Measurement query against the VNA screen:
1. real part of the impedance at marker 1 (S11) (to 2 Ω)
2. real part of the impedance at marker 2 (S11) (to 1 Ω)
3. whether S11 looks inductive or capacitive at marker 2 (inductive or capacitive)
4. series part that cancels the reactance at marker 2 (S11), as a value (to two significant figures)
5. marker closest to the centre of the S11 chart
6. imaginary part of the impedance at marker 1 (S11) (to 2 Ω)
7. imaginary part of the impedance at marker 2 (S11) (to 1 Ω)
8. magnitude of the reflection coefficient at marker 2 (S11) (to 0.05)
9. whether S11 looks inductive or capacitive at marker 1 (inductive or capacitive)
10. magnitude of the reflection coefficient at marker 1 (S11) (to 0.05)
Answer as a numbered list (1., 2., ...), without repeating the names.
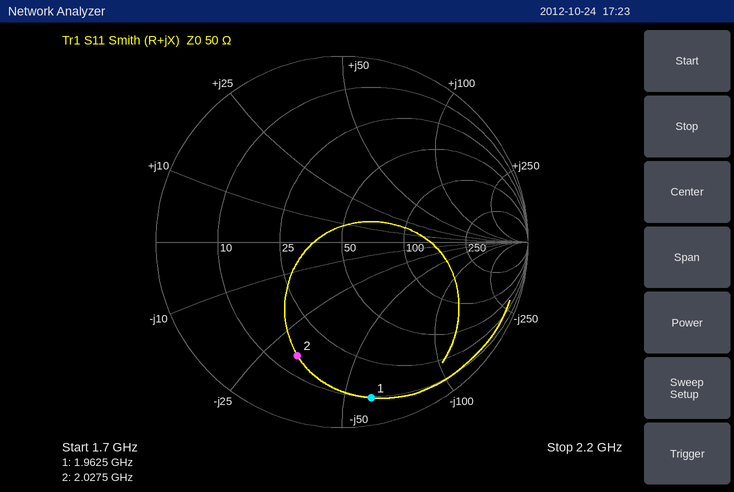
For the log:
1. 10 Ω
2. 15 Ω
3. capacitive
4. 2.5 nH
5. marker 2
6. -60 Ω
7. -32 Ω
8. 0.65
9. capacitive
10. 0.85
